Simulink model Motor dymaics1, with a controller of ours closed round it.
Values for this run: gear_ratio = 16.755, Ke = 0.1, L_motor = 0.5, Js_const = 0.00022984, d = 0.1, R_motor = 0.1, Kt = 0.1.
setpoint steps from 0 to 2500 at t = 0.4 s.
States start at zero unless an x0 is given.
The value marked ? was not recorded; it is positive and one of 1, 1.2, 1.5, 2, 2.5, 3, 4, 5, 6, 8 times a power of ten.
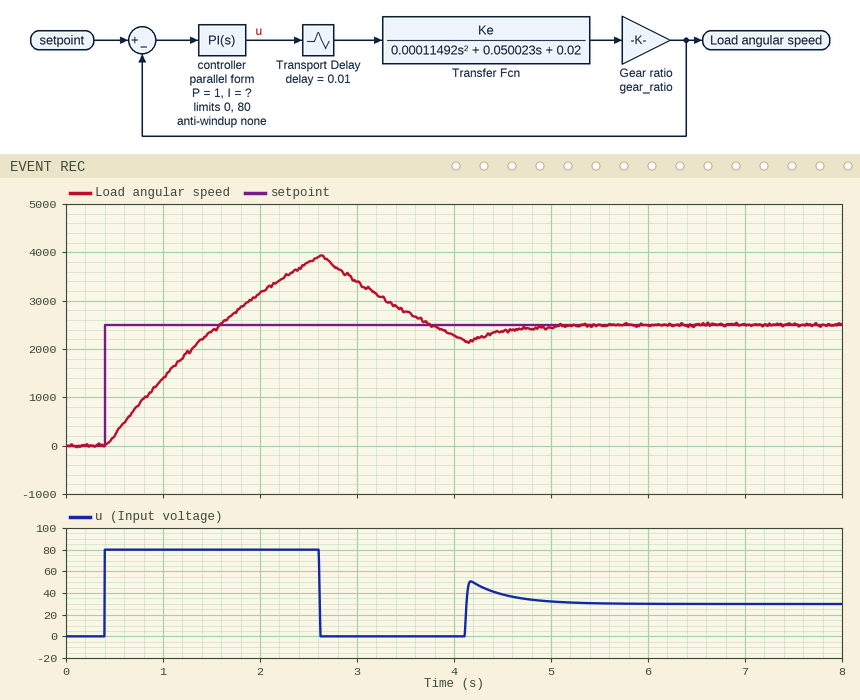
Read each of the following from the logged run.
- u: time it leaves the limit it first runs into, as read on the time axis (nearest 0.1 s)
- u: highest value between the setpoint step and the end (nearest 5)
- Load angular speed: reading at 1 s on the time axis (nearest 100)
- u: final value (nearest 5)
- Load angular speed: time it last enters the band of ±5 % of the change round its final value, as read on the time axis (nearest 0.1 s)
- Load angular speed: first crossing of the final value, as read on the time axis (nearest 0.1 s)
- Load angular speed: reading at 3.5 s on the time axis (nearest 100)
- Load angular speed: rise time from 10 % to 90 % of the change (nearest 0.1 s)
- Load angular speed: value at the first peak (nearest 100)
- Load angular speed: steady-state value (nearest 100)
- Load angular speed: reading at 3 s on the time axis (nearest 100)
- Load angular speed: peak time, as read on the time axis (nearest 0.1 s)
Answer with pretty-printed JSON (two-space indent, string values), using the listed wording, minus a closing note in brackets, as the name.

{
  "u: time it leaves the limit it first runs into, as read on the time axis": "2.6 s",
  "u: highest value between the setpoint step and the end": "80",
  "Load angular speed: reading at 1 s on the time axis": "1400",
  "u: final value": "30",
  "Load angular speed: time it last enters the band of ±5 % of the change round its final value, as read on the time axis": "4.5 s",
  "Load angular speed: first crossing of the final value, as read on the time axis": "1.6 s",
  "Load angular speed: reading at 3.5 s on the time axis": "2800",
  "Load angular speed: rise time from 10 % to 90 % of the change": "0.9 s",
  "Load angular speed: value at the first peak": "3900",
  "Load angular speed: steady-state value": "2500",
  "Load angular speed: reading at 3 s on the time axis": "3400",
  "Load angular speed: peak time, as read on the time axis": "2.6 s"
}
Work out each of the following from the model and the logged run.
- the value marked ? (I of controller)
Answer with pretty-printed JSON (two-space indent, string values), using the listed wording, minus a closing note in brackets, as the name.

{
  "the value marked ?": "2.5"
}
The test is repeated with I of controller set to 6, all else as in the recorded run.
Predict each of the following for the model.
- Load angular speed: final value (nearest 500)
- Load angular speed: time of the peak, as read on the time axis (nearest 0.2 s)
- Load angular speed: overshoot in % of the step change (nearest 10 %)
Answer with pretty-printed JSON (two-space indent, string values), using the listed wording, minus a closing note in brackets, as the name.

{
  "Load angular speed: final value": "2500",
  "Load angular speed: time of the peak, as read on the time axis": "2.8 s",
  "Load angular speed: overshoot in % of the step change": "70 %"
}
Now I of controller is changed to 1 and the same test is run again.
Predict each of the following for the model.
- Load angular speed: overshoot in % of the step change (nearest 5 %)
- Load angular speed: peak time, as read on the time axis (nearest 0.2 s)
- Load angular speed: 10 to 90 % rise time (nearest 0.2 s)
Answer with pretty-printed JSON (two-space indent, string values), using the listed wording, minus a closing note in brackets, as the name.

{
  "Load angular speed: overshoot in % of the step change": "40 %",
  "Load angular speed: peak time, as read on the time axis": "2.2 s",
  "Load angular speed: 10 to 90 % rise time": "1.0 s"
}
